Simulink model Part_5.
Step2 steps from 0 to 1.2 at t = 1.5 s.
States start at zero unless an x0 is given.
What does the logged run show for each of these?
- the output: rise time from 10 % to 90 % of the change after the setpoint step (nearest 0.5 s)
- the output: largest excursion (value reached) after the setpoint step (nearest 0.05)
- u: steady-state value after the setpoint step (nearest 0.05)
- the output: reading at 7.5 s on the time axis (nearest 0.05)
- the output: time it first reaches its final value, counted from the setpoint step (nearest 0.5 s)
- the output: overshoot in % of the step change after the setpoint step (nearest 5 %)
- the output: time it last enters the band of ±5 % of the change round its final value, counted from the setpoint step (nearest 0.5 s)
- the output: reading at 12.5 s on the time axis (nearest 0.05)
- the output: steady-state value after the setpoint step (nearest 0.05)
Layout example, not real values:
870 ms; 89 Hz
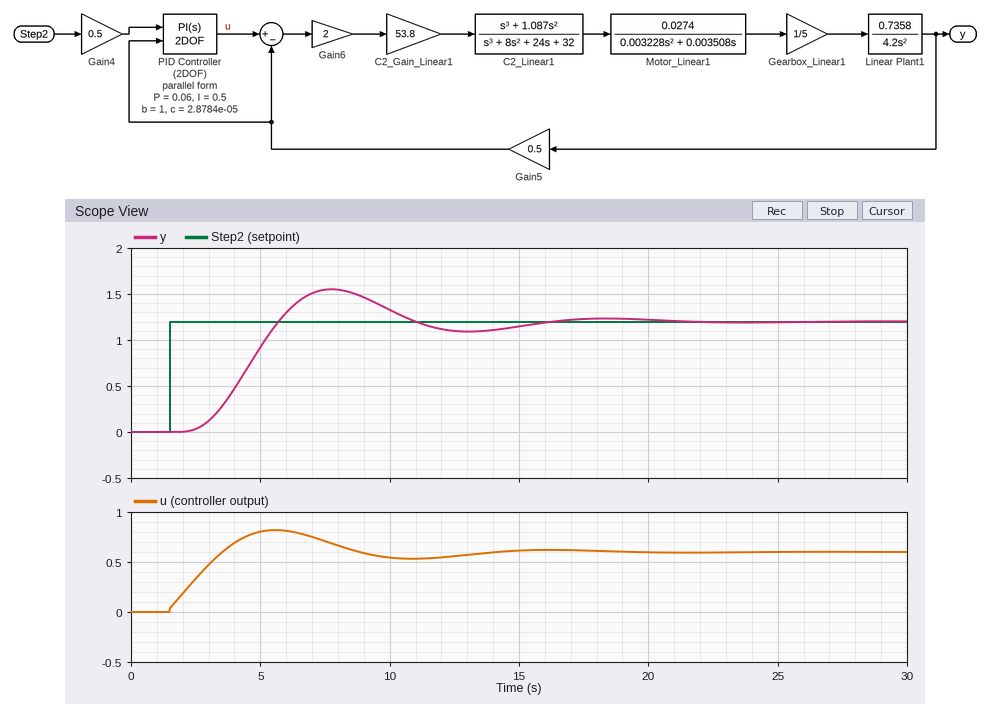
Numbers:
2.5 s; 1.55; 0.60; 1.55; 4.0 s; 30 %; 13.5 s; 1.10; 1.20
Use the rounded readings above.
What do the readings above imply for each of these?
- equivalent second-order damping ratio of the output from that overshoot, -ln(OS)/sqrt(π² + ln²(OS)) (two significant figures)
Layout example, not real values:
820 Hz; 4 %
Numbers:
0.36
